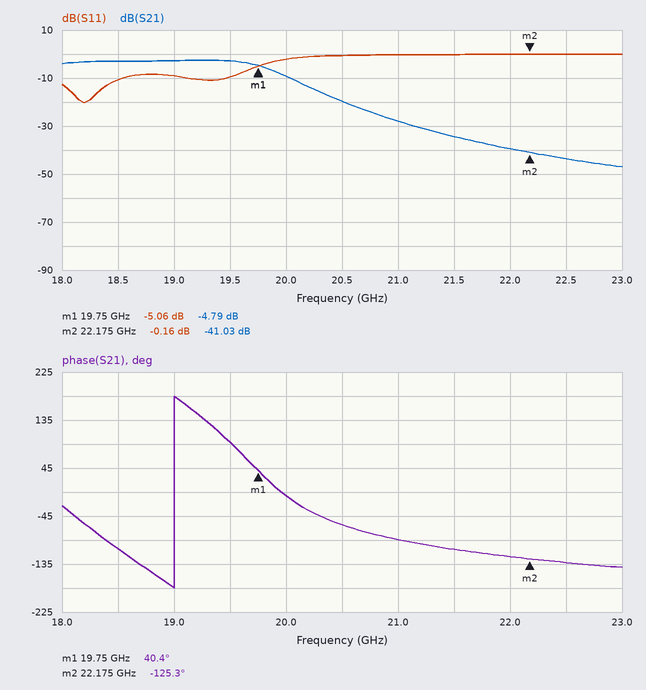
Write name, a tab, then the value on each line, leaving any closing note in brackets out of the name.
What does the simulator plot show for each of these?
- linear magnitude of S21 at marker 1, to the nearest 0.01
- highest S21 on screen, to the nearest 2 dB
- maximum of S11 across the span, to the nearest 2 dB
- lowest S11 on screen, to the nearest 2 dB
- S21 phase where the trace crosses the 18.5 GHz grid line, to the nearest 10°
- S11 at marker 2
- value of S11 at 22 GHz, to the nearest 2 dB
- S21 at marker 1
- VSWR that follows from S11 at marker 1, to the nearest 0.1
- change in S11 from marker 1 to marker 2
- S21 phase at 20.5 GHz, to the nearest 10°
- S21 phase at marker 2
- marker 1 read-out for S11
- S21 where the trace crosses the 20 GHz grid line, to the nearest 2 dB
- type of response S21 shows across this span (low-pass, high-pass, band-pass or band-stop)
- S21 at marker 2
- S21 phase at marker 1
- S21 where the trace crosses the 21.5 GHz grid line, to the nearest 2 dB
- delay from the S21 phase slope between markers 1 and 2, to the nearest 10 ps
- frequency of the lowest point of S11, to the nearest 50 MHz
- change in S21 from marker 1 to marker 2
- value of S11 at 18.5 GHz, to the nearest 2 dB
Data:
linear magnitude of S21 at marker 1, to the nearest 0.01	0.58
highest S21 on screen, to the nearest 2 dB	-2 dB
maximum of S11 across the span, to the nearest 2 dB	0 dB
lowest S11 on screen, to the nearest 2 dB	-20 dB
S21 phase where the trace crosses the 18.5 GHz grid line, to the nearest 10°	-110°
S11 at marker 2	-0.16 dB
value of S11 at 22 GHz, to the nearest 2 dB	0 dB
S21 at marker 1	-4.79 dB
VSWR that follows from S11 at marker 1, to the nearest 0.1	3.5
change in S11 from marker 1 to marker 2	4.90 dB
S21 phase at 20.5 GHz, to the nearest 10°	-60°
S21 phase at marker 2	-125.3°
marker 1 read-out for S11	-5.06 dB
S21 where the trace crosses the 20 GHz grid line, to the nearest 2 dB	-10 dB
type of response S21 shows across this span	low-pass
S21 at marker 2	-41.03 dB
S21 phase at marker 1	40.4°
S21 where the trace crosses the 21.5 GHz grid line, to the nearest 2 dB	-34 dB
delay from the S21 phase slope between markers 1 and 2, to the nearest 10 ps	190 ps
frequency of the lowest point of S11, to the nearest 50 MHz	18.20 GHz
change in S21 from marker 1 to marker 2	-36.24 dB
value of S11 at 18.5 GHz, to the nearest 2 dB	-10 dB
